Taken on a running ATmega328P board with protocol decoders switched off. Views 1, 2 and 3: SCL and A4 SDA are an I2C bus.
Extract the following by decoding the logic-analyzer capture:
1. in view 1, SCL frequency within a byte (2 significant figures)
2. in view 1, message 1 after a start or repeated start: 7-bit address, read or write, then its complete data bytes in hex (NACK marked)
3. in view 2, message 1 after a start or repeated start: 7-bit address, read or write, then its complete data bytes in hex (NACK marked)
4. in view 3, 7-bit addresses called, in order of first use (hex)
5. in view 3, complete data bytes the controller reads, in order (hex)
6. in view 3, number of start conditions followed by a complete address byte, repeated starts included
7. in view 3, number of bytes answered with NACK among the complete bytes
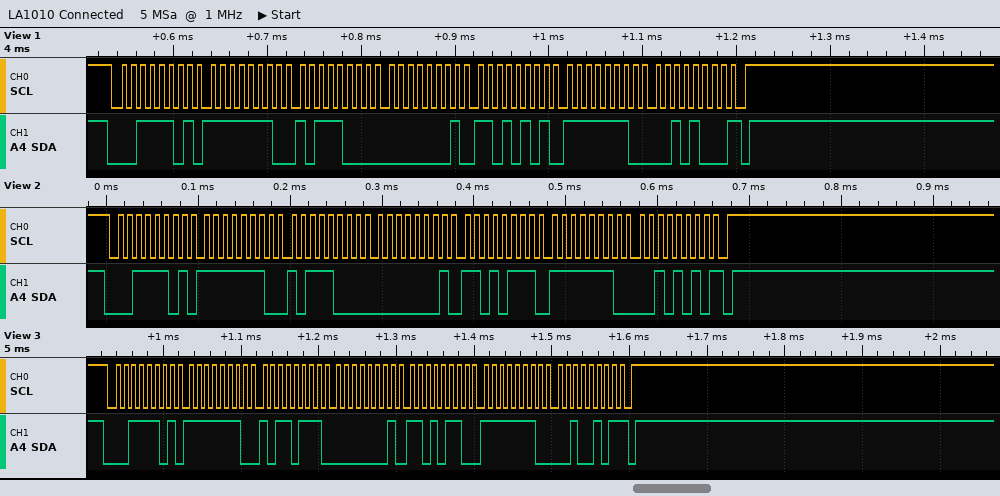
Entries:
100 kHz
0x1E read: FE B8 01 D5 FE 28 NACK
0x1E read: FE B8 01 D7 FE 2A NACK
0x1E
FE B7 01 D6 FE 25
1
1
